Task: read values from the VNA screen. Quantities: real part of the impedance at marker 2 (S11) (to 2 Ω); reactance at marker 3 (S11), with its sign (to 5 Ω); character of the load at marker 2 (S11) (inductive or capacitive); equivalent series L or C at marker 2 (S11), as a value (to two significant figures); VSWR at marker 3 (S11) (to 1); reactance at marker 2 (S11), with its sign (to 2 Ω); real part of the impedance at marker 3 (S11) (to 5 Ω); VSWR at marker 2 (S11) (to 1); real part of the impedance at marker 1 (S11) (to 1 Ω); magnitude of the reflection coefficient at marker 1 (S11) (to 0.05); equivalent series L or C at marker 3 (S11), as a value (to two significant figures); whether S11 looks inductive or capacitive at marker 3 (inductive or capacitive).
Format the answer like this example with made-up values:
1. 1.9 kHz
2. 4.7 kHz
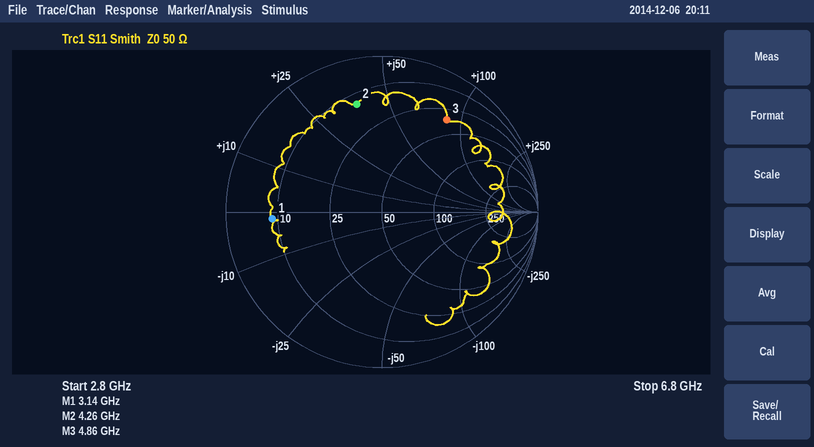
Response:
1. 14 Ω
2. +85 Ω
3. inductive
4. 1.4 nH
5. 6
6. +38 Ω
7. 35 Ω
8. 6
9. 9 Ω
10. 0.70
11. 2.8 nH
12. inductive
